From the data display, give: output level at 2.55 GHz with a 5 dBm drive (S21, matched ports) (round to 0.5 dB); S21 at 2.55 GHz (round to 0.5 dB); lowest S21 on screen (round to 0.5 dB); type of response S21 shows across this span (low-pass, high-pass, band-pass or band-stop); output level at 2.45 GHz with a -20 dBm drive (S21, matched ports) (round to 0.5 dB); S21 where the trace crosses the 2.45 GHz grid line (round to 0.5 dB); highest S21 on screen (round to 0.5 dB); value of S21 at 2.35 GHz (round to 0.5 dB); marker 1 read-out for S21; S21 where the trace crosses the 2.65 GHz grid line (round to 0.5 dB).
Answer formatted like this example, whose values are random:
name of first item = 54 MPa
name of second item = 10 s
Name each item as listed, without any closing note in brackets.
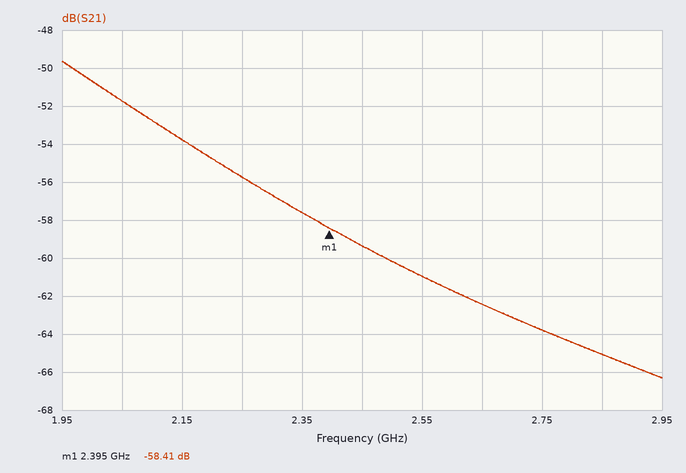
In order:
output level at 2.55 GHz with a 5 dBm drive (S21, matched ports) = -56.0 dBm
S21 at 2.55 GHz = -61.0 dB
lowest S21 on screen = -66.5 dB
type of response S21 shows across this span = low-pass
output level at 2.45 GHz with a -20 dBm drive (S21, matched ports) = -79.5 dBm
S21 where the trace crosses the 2.45 GHz grid line = -59.5 dB
highest S21 on screen = -49.5 dB
value of S21 at 2.35 GHz = -57.5 dB
marker 1 read-out for S21 = -58.41 dB
S21 where the trace crosses the 2.65 GHz grid line = -62.5 dB
